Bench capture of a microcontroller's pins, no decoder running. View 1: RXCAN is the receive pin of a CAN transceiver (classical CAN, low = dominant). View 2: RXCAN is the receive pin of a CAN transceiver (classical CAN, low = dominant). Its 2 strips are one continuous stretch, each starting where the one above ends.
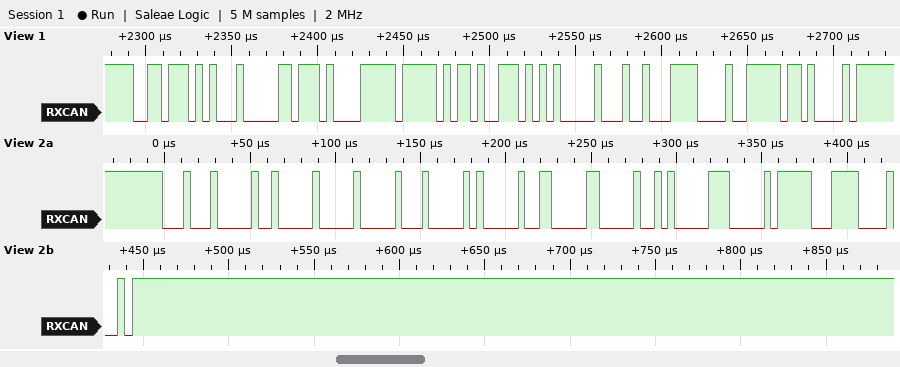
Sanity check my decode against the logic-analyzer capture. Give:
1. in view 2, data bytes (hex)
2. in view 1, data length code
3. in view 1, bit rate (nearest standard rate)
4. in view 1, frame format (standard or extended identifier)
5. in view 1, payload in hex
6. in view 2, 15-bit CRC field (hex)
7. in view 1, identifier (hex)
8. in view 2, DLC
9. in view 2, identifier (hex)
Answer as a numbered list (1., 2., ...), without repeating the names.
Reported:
1. 00 01 02 03 04 05 06 07
2. 8
3. 250 kbit/s
4. standard
5. 2E 87 FF 69 D5 00 91 E1
6. 0x6784
7. 0x375
8. 8
9. 0x110
